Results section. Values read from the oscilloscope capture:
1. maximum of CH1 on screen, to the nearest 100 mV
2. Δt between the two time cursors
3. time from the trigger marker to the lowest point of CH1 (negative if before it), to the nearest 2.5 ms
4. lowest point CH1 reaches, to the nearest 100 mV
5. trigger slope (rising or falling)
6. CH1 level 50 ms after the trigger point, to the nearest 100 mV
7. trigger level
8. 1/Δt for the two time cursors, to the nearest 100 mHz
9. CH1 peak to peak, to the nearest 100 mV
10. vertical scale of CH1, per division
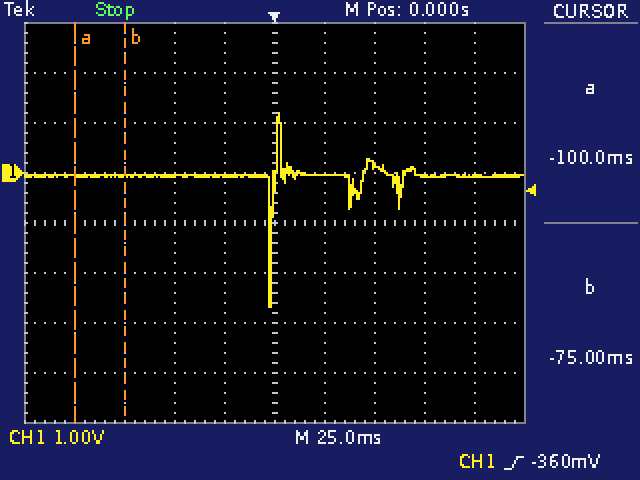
1.2 V
25.0 ms
-2.5 ms
-2.7 V
rising
200 mV
-360 mV
40.0 Hz
3.9 V
1 V
